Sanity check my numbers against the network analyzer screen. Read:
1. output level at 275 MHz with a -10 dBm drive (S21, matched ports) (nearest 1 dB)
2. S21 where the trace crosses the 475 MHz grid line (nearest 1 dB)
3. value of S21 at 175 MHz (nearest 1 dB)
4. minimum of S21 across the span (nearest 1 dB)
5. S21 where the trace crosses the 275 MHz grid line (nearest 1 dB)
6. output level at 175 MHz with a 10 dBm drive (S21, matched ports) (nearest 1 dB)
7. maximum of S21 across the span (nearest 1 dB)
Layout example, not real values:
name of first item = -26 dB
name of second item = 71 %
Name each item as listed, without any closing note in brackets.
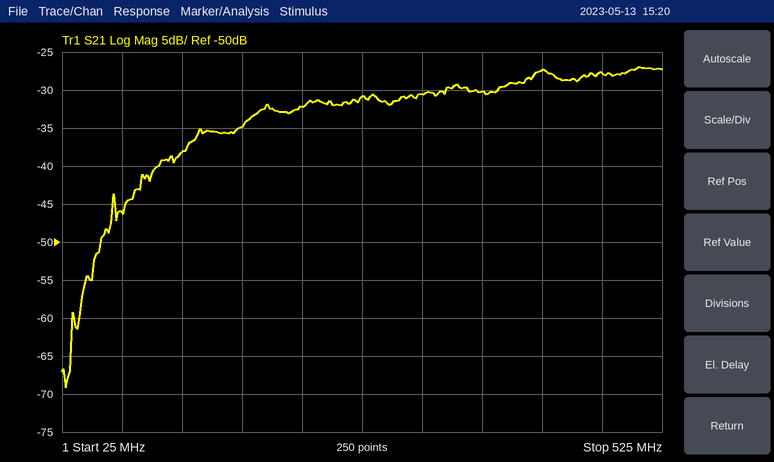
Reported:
output level at 275 MHz with a -10 dBm drive (S21, matched ports) = -41 dBm
S21 where the trace crosses the 475 MHz grid line = -28 dB
value of S21 at 175 MHz = -35 dB
minimum of S21 across the span = -69 dB
S21 where the trace crosses the 275 MHz grid line = -31 dB
output level at 175 MHz with a 10 dBm drive (S21, matched ports) = -25 dBm
maximum of S21 across the span = -27 dB
